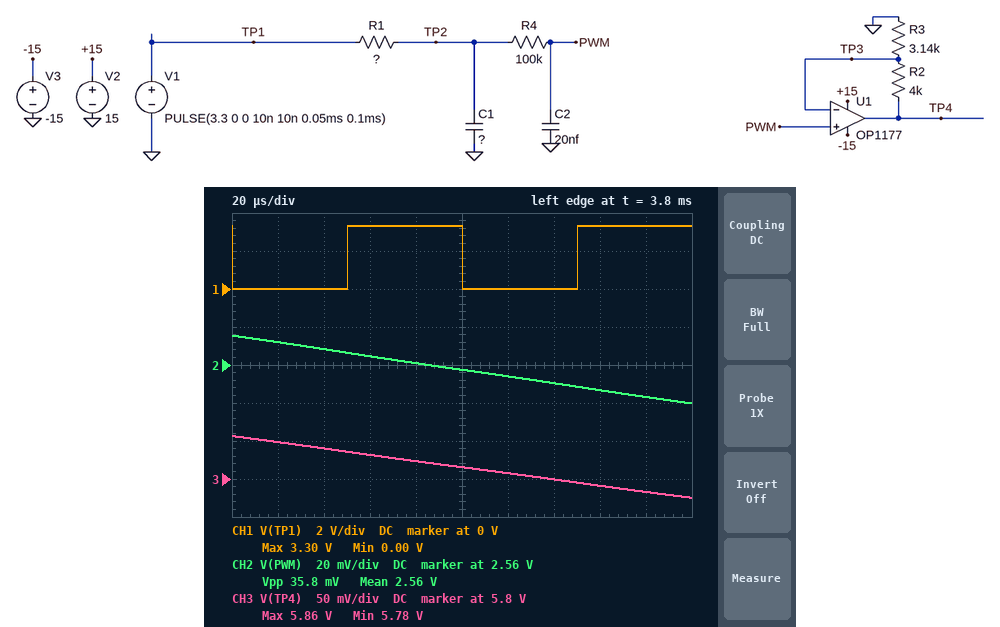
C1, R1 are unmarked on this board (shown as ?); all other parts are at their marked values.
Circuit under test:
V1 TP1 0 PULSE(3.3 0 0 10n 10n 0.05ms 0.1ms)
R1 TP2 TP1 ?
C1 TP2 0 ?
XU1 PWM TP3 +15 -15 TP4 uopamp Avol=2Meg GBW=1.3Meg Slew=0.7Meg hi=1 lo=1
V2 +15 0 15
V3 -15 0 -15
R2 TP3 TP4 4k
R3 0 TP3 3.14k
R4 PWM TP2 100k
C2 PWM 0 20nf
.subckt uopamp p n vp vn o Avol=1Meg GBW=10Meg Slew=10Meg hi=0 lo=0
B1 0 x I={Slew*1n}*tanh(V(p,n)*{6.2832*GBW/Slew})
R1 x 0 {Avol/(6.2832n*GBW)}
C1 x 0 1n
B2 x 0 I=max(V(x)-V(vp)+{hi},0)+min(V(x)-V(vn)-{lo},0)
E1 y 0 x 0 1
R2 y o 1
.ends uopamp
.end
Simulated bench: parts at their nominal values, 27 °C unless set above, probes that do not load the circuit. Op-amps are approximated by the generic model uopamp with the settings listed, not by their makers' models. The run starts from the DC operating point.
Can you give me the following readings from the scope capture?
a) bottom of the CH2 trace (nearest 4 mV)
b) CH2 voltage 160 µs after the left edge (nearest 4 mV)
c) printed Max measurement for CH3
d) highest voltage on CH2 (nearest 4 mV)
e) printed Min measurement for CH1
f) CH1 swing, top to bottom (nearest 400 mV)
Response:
2.540 V
2.548 V
5.86 V
2.576 V
0.00 V
3.2 V
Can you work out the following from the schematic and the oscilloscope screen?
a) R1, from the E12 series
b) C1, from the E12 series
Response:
82 kΩ
27 nF
